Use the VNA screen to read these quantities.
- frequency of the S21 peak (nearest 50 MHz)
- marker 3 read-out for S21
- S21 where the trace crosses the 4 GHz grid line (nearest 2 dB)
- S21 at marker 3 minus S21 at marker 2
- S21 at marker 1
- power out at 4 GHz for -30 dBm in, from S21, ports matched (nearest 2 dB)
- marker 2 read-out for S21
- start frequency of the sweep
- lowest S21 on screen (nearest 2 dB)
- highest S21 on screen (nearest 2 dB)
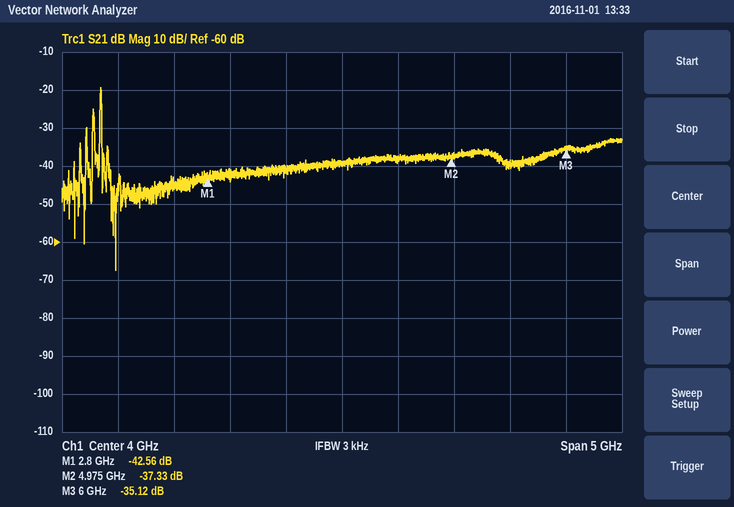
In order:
1.85 GHz
-35.12 dB
-40 dB
2.21 dB
-42.56 dB
-70 dBm
-37.33 dB
1.5 GHz
-68 dB
-20 dB
